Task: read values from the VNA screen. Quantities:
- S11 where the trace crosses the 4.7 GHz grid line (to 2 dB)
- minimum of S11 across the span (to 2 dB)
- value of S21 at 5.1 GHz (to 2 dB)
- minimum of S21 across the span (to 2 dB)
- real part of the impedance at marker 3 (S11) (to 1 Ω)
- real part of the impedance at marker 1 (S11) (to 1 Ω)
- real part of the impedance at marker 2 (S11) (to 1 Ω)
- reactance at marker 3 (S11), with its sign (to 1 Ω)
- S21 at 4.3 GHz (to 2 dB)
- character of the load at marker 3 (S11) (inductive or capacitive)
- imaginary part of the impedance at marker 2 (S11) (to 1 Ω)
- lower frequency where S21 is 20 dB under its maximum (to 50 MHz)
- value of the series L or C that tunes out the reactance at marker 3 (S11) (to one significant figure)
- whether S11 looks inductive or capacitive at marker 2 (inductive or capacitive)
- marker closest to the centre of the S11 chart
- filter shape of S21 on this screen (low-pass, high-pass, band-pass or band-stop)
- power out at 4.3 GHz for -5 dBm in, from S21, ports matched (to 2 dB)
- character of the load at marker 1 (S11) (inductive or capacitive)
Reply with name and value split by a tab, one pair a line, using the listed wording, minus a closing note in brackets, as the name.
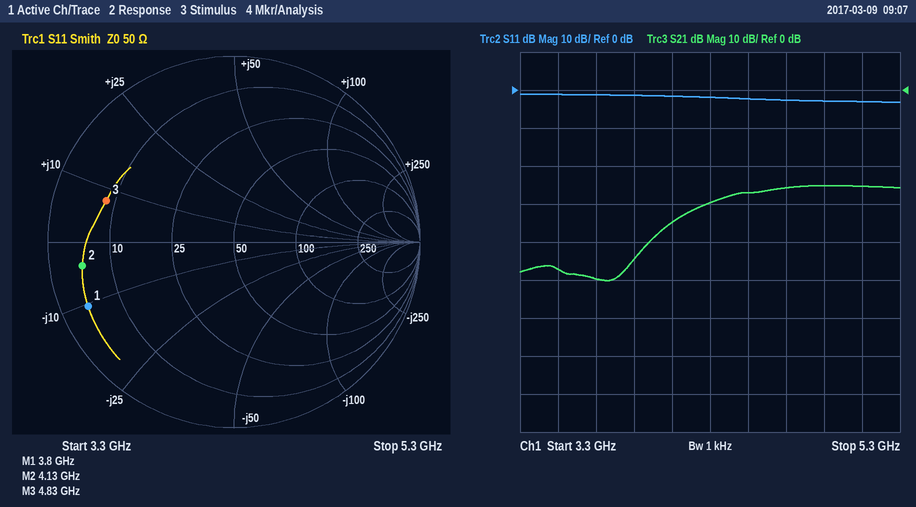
S11 where the trace crosses the 4.7 GHz grid line	-2 dB
minimum of S11 across the span	-4 dB
value of S21 at 5.1 GHz	-26 dB
minimum of S21 across the span	-50 dB
real part of the impedance at marker 3 (S11)	8 Ω
real part of the impedance at marker 1 (S11)	4 Ω
real part of the impedance at marker 2 (S11)	5 Ω
reactance at marker 3 (S11), with its sign	+8 Ω
S21 at 4.3 GHz	-30 dB
character of the load at marker 3 (S11)	inductive
imaginary part of the impedance at marker 2 (S11)	-4 Ω
lower frequency where S21 is 20 dB under its maximum	3.90 GHz
value of the series L or C that tunes out the reactance at marker 3 (S11)	4 pF
whether S11 looks inductive or capacitive at marker 2	capacitive
marker closest to the centre of the S11 chart	marker 3
filter shape of S21 on this screen	high-pass
power out at 4.3 GHz for -5 dBm in, from S21, ports matched	-34 dBm
character of the load at marker 1 (S11)	capacitive
